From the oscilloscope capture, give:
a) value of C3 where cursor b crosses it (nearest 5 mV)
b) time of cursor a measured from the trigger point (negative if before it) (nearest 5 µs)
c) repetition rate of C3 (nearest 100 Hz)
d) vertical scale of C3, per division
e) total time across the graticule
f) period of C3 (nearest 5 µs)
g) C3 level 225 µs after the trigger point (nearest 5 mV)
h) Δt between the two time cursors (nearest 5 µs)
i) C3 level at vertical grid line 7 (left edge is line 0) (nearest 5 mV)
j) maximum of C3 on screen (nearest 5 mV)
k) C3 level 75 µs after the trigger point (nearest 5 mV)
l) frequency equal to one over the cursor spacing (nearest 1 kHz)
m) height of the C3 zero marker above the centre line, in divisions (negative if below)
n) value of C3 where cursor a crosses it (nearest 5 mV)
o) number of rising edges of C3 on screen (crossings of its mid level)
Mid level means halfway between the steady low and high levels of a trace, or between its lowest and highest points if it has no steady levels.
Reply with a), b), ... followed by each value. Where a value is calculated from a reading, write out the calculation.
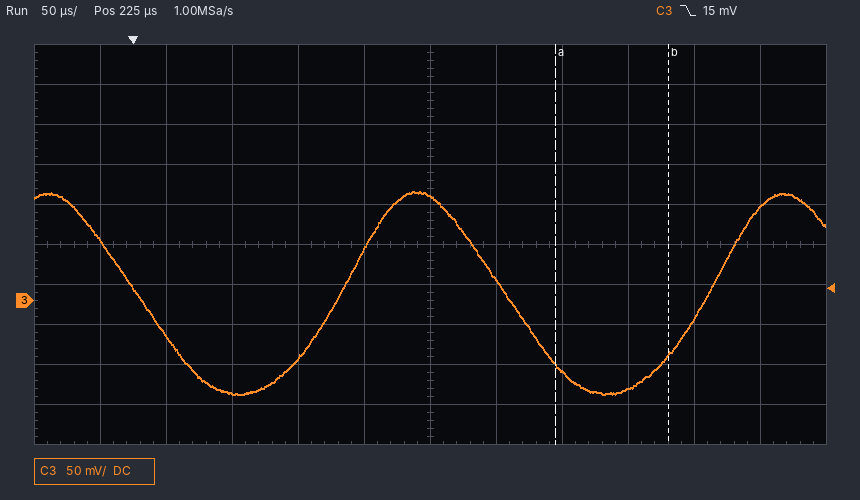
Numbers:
a) -70 mV
b) +320 µs
c) 1 / 280 µs ≈ 3.6 kHz
d) 50 mV
e) 600 µs
f) 280 µs
g) 130 mV
h) 85 µs
i) 25 mV
j) 135 mV
k) -115 mV
l) 1 / 85 µs ≈ 12 kHz
m) -1.4 div
n) -80 mV
o) 2
